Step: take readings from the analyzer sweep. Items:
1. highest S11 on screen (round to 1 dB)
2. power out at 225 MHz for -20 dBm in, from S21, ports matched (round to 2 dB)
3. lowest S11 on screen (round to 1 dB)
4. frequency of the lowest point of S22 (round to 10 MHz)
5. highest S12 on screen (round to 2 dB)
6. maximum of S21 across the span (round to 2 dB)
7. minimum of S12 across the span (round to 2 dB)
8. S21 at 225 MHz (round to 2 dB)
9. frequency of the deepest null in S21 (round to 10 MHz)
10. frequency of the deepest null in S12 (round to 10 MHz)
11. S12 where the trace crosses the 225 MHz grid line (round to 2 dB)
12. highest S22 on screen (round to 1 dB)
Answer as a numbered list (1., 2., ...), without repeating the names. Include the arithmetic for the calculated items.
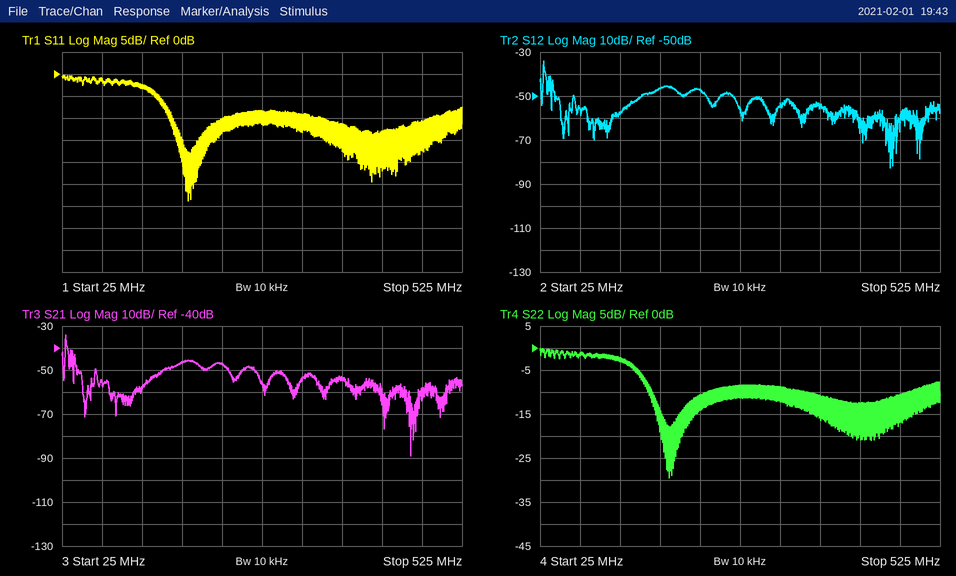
1. 0 dB
2. -20 dBm + (-48 dB) = -68 dBm
3. -29 dB
4. 190 MHz
5. -34 dB
6. -34 dB
7. -82 dB
8. -48 dB
9. 460 MHz
10. 460 MHz
11. -48 dB
12. 0 dB
